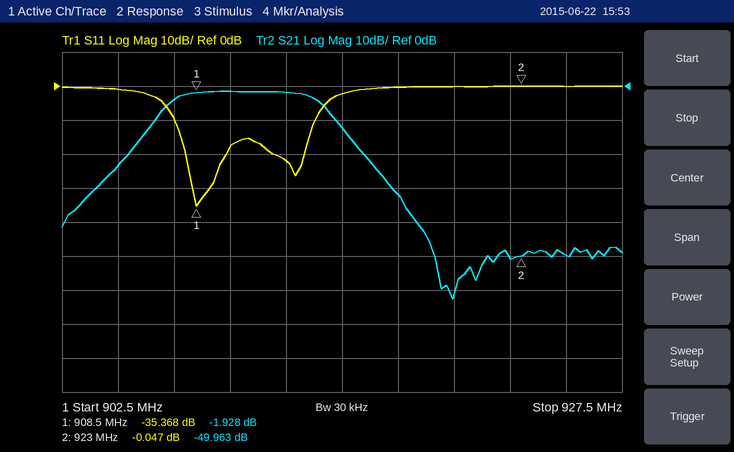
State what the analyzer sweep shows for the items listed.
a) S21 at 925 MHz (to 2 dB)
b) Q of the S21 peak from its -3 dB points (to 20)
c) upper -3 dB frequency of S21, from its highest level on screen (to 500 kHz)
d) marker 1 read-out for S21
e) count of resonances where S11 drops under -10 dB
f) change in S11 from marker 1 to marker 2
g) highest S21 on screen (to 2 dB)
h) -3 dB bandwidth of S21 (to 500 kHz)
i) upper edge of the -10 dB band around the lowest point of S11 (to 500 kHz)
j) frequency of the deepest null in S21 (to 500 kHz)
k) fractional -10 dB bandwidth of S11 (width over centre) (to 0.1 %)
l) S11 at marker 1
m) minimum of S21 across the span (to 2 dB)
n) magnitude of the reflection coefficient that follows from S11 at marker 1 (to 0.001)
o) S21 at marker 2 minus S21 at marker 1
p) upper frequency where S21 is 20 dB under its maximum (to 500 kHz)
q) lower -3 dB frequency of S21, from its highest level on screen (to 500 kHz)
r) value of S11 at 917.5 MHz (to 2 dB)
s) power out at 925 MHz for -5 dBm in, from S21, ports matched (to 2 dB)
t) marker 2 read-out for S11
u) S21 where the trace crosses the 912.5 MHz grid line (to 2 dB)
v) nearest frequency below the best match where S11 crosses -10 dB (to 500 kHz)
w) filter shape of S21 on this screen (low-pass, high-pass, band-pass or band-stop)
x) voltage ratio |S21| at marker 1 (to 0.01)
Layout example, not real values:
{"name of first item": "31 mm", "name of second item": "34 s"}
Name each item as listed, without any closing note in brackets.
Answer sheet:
{"S21 at 925 MHz": "-50 dB", "Q of the S21 peak from its -3 dB points": "140", "upper -3 dB frequency of S21, from its highest level on screen": "914.0 MHz", "marker 1 read-out for S21": "-1.928 dB", "count of resonances where S11 drops under -10 dB": "2", "change in S11 from marker 1 to marker 2": "35.321 dB", "highest S21 on screen": "-2 dB", "-3 dB bandwidth of S21": "6.5 MHz", "upper edge of the -10 dB band around the lowest point of S11": "914.0 MHz", "frequency of the deepest null in S21": "920.0 MHz", "fractional -10 dB bandwidth of S11 (width over centre)": "0.7 %", "S11 at marker 1": "-35.368 dB", "minimum of S21 across the span": "-62 dB", "magnitude of the reflection coefficient that follows from S11 at marker 1": "0.017", "S21 at marker 2 minus S21 at marker 1": "-48.035 dB", "upper frequency where S21 is 20 dB under its maximum": "916.0 MHz", "lower -3 dB frequency of S21, from its highest level on screen": "907.5 MHz", "value of S11 at 917.5 MHz": "0 dB", "power out at 925 MHz for -5 dBm in, from S21, ports matched": "-54 dBm", "marker 2 read-out for S11": "-0.047 dB", "S21 where the trace crosses the 912.5 MHz grid line": "-2 dB", "nearest frequency below the best match where S11 crosses -10 dB": "907.5 MHz", "filter shape of S21 on this screen": "band-pass", "voltage ratio |S21| at marker 1": "0.80"}
